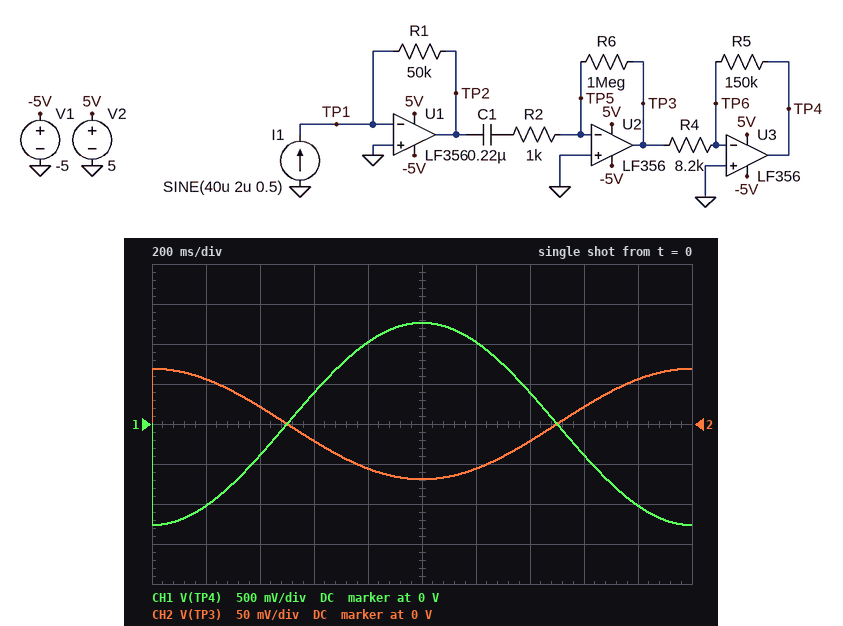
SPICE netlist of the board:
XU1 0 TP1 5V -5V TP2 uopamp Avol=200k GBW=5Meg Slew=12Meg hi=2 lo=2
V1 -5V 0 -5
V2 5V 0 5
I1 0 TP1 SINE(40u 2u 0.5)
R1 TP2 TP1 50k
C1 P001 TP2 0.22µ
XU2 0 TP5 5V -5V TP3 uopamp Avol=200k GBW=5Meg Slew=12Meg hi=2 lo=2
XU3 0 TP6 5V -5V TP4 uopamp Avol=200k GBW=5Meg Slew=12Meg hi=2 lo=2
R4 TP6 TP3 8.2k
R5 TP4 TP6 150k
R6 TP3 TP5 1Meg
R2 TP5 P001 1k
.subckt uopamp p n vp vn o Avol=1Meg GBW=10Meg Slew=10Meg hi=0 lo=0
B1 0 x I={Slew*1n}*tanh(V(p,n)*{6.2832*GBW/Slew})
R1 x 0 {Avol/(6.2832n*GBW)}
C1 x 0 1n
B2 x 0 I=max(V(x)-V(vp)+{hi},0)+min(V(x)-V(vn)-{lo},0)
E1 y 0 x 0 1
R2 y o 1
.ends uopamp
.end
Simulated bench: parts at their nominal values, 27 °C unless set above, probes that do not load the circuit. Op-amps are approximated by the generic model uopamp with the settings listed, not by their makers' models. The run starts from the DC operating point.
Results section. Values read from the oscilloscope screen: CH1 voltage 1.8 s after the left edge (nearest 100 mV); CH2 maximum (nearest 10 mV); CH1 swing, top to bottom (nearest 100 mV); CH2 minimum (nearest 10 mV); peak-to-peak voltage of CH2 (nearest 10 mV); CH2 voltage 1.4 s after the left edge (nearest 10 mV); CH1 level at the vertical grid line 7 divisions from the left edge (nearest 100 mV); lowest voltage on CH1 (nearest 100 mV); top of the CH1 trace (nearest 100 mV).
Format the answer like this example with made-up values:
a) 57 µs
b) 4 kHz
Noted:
a) -1.0 V
b) 70 mV
c) 2.5 V
d) -70 mV
e) 140 mV
f) -20 mV
g) 400 mV
h) -1.3 V
i) 1.3 V
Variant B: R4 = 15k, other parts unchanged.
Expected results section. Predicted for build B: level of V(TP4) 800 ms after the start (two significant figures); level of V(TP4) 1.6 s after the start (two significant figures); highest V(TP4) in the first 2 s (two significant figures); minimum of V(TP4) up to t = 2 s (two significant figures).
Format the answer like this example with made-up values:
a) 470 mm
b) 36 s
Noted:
a) 560 mV
b) -210 mV
c) 690 mV
d) -690 mV
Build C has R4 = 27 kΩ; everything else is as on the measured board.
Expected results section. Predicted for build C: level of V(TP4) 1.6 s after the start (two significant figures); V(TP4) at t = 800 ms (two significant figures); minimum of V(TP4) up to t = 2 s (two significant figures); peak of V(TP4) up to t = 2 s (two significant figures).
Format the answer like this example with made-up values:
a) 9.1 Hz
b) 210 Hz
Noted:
a) -120 mV
b) 310 mV
c) -380 mV
d) 380 mV
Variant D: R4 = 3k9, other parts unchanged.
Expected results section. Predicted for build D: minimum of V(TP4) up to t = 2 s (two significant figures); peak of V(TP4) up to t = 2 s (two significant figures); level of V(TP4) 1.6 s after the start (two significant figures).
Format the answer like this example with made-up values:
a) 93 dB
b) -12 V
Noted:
a) -2.7 V
b) 2.7 V
c) -820 mV
